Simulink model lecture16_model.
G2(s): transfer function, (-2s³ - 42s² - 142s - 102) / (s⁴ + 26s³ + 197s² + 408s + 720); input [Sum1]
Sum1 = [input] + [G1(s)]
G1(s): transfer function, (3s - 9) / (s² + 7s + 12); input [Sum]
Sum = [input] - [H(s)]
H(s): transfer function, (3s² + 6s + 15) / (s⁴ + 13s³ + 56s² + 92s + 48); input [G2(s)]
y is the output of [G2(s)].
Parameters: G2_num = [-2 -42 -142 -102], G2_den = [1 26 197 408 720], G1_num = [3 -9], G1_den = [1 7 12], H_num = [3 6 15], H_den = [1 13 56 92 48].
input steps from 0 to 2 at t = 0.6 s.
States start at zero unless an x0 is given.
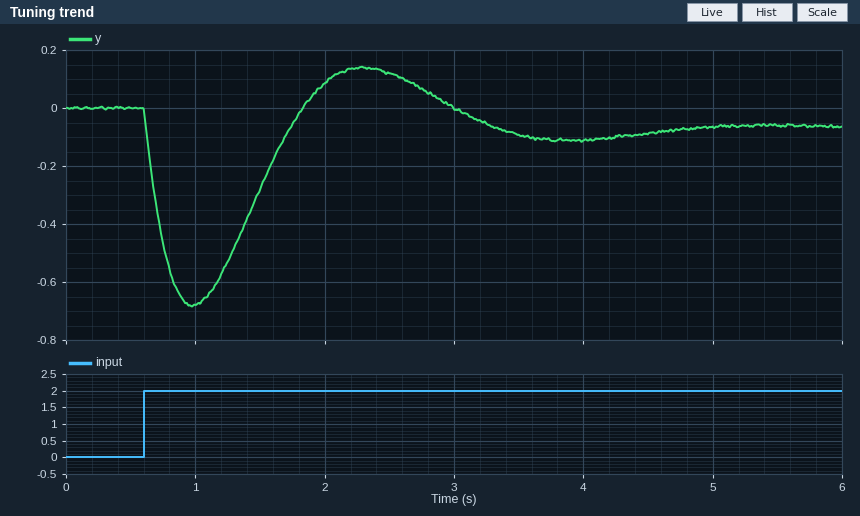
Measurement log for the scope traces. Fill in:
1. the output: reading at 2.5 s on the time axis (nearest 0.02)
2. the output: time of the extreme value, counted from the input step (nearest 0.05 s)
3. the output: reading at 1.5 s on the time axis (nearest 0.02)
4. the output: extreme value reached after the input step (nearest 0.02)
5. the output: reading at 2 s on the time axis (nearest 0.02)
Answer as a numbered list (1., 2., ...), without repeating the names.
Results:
1. 0.12
2. 0.40 s
3. -0.28
4. -0.68
5. 0.08
